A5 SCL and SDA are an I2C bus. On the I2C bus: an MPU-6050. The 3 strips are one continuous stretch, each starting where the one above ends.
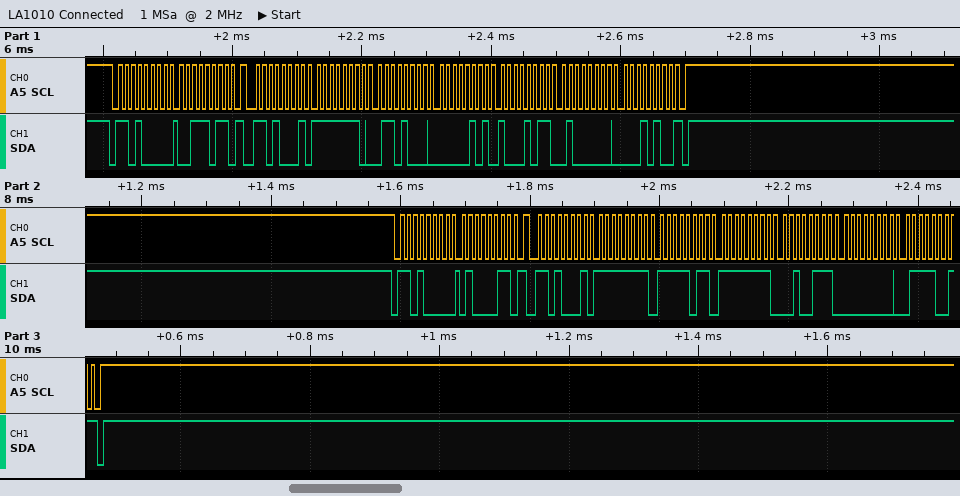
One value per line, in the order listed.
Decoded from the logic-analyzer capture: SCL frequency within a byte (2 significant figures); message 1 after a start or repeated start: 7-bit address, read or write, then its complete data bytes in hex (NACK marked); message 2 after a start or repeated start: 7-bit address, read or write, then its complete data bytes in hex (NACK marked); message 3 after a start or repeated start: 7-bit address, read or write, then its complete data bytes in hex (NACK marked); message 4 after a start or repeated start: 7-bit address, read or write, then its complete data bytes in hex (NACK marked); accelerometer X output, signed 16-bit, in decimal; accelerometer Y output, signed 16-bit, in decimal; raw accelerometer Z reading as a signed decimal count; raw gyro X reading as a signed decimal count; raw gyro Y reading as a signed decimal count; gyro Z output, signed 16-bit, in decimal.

100 kHz
0x68 write: 3B
0x68 read: FE 68 05 8B 40 14 NACK
0x68 write: 43
0x68 read: FF FB FF 27 00 79 NACK
-408
1419
16404
-5
-217
121
